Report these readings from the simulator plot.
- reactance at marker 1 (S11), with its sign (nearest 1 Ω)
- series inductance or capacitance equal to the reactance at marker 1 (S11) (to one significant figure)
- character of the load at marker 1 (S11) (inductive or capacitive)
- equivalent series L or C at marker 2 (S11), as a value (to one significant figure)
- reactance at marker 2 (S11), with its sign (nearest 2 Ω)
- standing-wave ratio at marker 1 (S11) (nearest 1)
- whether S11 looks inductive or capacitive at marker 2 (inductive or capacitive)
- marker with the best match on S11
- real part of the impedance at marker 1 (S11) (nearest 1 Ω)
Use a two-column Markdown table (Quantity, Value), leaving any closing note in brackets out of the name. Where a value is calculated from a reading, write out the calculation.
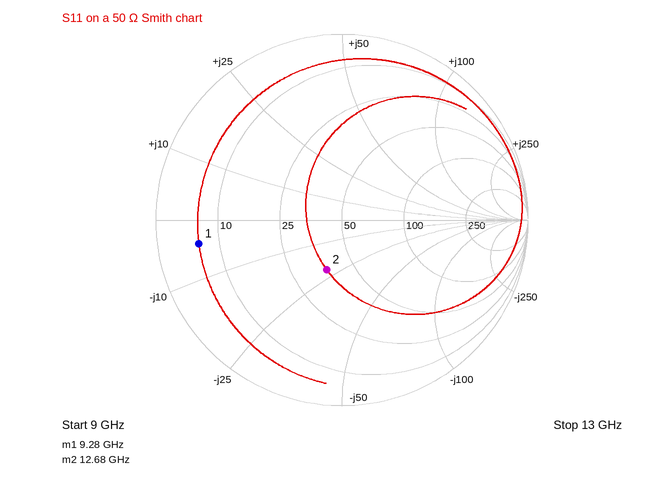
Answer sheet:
| Quantity | Value |
|---|---|
| reactance at marker 1 (S11), with its sign | -4 Ω |
| series inductance or capacitance equal to the reactance at marker 1 (S11) | C = 1/(2π × 9.28 GHz × 4 Ω) ≈ 4 pF |
| character of the load at marker 1 (S11) | capacitive |
| equivalent series L or C at marker 2 (S11), as a value | C = 1/(2π × 12.68 GHz × 22 Ω) ≈ 571 fF, so 600 fF to one significant figure |
| reactance at marker 2 (S11), with its sign | -22 Ω |
| standing-wave ratio at marker 1 (S11) | 8 |
| whether S11 looks inductive or capacitive at marker 2 | capacitive |
| marker with the best match on S11 | marker 2 |
| real part of the impedance at marker 1 (S11) | 6 Ω |
